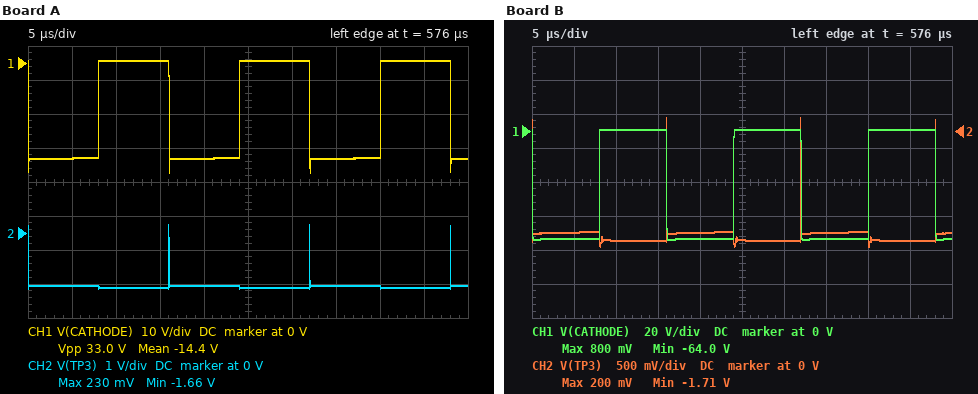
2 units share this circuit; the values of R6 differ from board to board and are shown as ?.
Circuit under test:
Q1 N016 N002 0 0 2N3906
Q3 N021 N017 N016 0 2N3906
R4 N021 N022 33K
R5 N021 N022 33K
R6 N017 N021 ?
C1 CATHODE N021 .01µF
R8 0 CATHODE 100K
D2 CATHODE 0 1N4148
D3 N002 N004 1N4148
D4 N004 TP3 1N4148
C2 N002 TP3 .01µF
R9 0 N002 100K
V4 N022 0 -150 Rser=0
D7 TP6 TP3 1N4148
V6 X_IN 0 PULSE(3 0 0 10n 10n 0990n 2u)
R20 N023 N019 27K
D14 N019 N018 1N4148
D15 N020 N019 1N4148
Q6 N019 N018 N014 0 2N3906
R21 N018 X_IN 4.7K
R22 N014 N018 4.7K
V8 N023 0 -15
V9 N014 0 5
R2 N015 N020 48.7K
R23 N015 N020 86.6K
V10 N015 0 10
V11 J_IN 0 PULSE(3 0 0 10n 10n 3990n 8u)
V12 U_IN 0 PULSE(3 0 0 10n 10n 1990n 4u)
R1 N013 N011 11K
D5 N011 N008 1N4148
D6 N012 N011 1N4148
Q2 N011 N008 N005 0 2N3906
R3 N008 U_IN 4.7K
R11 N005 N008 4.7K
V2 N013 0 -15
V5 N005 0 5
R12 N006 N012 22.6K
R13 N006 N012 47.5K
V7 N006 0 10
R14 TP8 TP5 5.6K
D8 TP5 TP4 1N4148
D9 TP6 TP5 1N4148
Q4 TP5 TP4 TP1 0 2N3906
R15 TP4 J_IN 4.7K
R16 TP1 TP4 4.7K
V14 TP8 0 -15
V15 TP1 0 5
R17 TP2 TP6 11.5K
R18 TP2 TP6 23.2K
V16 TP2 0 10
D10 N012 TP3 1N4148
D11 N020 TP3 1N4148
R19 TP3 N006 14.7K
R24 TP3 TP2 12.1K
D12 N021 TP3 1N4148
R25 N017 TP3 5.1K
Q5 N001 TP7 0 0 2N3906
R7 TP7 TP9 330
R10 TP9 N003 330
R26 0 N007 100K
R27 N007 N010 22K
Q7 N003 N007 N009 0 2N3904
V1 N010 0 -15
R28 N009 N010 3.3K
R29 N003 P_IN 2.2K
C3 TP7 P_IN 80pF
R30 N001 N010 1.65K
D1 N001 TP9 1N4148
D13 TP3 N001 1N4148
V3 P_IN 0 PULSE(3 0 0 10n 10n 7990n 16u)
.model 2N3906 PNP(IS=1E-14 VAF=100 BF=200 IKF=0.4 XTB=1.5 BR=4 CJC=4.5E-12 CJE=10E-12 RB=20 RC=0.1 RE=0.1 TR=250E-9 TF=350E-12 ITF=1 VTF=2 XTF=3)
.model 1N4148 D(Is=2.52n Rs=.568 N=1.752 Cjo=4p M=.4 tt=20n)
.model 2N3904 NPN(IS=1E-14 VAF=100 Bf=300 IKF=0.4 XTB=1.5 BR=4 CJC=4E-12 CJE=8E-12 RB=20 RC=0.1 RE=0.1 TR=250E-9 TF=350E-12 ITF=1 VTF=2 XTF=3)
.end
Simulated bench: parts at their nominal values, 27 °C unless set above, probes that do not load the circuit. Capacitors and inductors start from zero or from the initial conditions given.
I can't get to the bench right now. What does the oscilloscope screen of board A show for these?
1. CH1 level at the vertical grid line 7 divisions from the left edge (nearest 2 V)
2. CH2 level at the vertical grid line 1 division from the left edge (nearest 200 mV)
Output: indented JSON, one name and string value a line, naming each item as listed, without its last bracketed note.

{
  "CH1 level at the vertical grid line 7 divisions from the left edge": "-28 V",
  "CH2 level at the vertical grid line 1 division from the left edge": "-1.6 V"
}
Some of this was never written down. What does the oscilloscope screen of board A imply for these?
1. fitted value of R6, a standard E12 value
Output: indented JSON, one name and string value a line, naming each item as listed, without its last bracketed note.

{
  "fitted value of R6, a standard E12 value": "1.5 kΩ"
}
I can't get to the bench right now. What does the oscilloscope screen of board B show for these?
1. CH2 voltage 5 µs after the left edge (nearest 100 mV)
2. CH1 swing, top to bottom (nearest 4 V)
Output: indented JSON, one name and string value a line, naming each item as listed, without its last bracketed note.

{
  "CH2 voltage 5 µs after the left edge": "-1.5 V",
  "CH1 swing, top to bottom": "64 V"
}
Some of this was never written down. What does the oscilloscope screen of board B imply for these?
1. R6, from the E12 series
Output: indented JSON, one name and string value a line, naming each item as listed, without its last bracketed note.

{
  "R6, from the E12 series": "10 kΩ"
}
